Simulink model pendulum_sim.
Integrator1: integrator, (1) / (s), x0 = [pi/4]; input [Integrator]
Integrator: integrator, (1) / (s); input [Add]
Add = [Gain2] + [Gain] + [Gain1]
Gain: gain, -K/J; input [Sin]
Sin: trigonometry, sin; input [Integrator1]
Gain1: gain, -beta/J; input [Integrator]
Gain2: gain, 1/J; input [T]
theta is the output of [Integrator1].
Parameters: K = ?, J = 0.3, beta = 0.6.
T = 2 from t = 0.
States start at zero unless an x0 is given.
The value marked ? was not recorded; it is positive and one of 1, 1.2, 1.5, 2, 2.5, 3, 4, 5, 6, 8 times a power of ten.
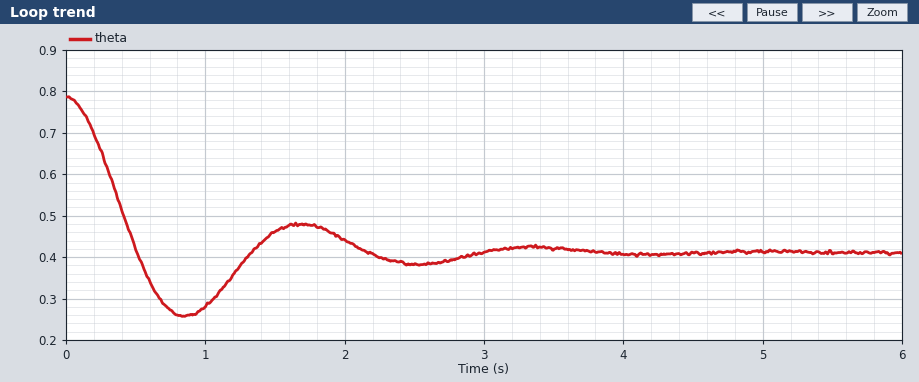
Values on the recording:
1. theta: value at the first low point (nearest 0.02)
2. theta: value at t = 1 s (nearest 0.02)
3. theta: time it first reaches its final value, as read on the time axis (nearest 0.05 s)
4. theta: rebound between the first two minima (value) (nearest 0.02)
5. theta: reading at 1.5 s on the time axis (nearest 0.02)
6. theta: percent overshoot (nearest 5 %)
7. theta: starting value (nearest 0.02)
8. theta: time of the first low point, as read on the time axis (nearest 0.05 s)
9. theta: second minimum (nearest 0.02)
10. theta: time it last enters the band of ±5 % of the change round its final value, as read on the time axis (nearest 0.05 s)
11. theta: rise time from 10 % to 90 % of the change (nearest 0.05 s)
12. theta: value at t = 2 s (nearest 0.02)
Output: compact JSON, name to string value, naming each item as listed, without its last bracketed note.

{"theta: value at the first low point": "0.26", "theta: value at t = 1 s": "0.28", "theta: time it first reaches its final value, as read on the time axis": "0.50 s", "theta: rebound between the first two minima (value)": "0.48", "theta: reading at 1.5 s on the time axis": "0.46", "theta: percent overshoot": "40 %", "theta: starting value": "0.78", "theta: time of the first low point, as read on the time axis": "0.85 s", "theta: second minimum": "0.38", "theta: time it last enters the band of ±5 % of the change round its final value, as read on the time axis": "2.75 s", "theta: rise time from 10 % to 90 % of the change": "0.35 s", "theta: value at t = 2 s": "0.44"}
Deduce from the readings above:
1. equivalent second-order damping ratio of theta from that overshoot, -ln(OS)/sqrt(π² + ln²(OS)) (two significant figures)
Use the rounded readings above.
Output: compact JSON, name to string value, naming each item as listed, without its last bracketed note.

{"equivalent second-order damping ratio of theta from that overshoot, -ln(OS)/sqrt(π² + ln²(OS))": "0.28"}
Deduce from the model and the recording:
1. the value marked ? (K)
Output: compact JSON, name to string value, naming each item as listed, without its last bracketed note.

{"the value marked ?": "5"}
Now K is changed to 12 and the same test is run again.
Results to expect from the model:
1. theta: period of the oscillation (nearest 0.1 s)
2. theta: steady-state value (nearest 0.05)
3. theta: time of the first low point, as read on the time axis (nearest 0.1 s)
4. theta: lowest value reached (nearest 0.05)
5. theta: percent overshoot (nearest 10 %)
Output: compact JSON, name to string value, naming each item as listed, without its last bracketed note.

{"theta: period of the oscillation": "1.0 s", "theta: steady-state value": "0.15", "theta: time of the first low point, as read on the time axis": "0.5 s", "theta: lowest value reached": "-0.20", "theta: percent overshoot": "60 %"}
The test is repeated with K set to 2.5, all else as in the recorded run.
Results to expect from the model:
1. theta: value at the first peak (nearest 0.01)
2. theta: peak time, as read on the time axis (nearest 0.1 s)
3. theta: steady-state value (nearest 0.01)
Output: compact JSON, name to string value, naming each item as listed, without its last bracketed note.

{"theta: value at the first peak": "0.96", "theta: peak time, as read on the time axis": "1.5 s", "theta: steady-state value": "0.93"}
